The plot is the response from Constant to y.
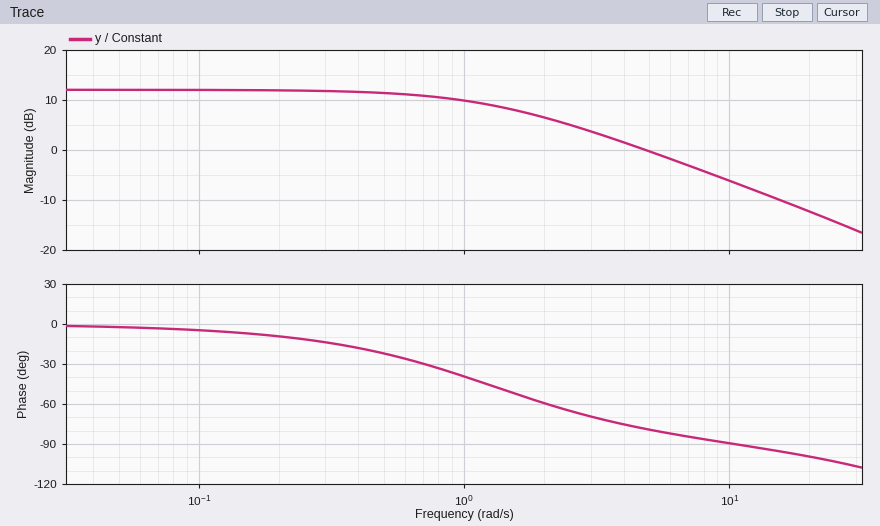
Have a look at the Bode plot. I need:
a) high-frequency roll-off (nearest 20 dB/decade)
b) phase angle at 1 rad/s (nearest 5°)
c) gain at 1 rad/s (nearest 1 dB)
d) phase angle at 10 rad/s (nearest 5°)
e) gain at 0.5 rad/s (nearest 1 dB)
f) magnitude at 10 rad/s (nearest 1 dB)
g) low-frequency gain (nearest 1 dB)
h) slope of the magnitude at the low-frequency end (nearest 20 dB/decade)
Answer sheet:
-20 dB/decade
-40°
10 dB
-90°
11 dB
-6 dB
12 dB
0 dB/decade
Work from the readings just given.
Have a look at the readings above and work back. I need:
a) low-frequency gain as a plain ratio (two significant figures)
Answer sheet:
4.0
